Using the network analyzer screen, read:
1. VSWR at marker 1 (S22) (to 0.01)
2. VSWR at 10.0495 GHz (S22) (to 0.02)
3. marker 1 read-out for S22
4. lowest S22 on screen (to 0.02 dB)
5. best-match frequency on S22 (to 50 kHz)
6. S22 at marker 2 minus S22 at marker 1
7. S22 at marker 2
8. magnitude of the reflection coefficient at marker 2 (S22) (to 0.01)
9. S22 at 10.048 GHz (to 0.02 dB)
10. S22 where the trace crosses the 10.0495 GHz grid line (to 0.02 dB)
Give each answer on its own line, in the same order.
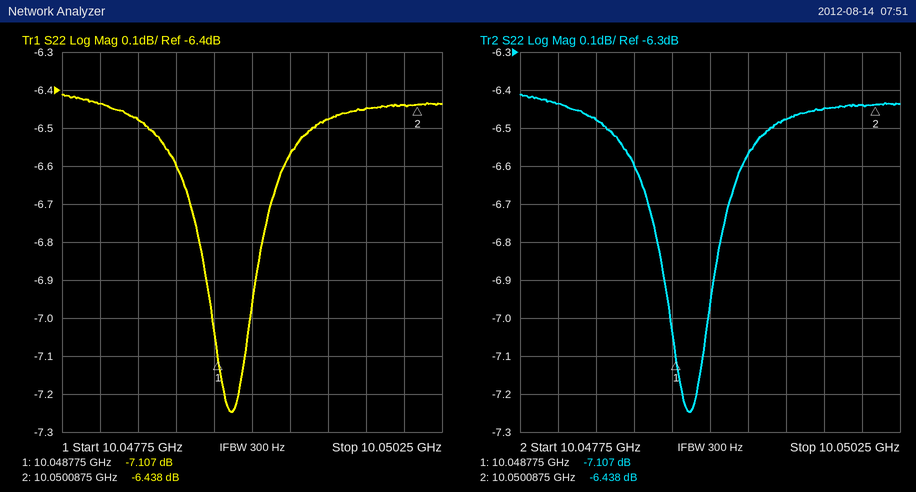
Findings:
2.58
2.80
-7.107 dB
-7.24 dB
10.04885 GHz
0.669 dB
-6.438 dB
0.48
-6.44 dB
-6.48 dB
